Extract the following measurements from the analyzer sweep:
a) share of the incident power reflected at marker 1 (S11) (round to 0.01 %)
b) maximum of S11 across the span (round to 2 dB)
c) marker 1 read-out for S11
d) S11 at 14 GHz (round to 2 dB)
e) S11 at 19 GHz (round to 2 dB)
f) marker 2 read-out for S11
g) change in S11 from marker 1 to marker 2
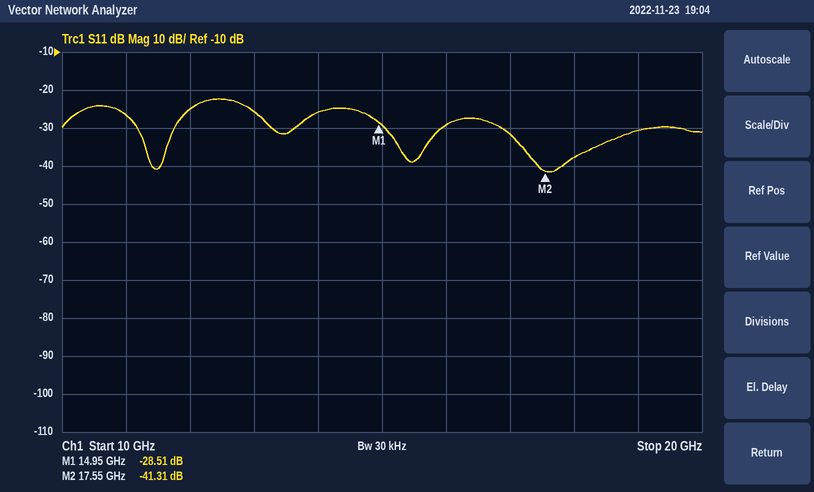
0.14 %
-22 dB
-28.51 dB
-26 dB
-30 dB
-41.31 dB
-12.80 dB
